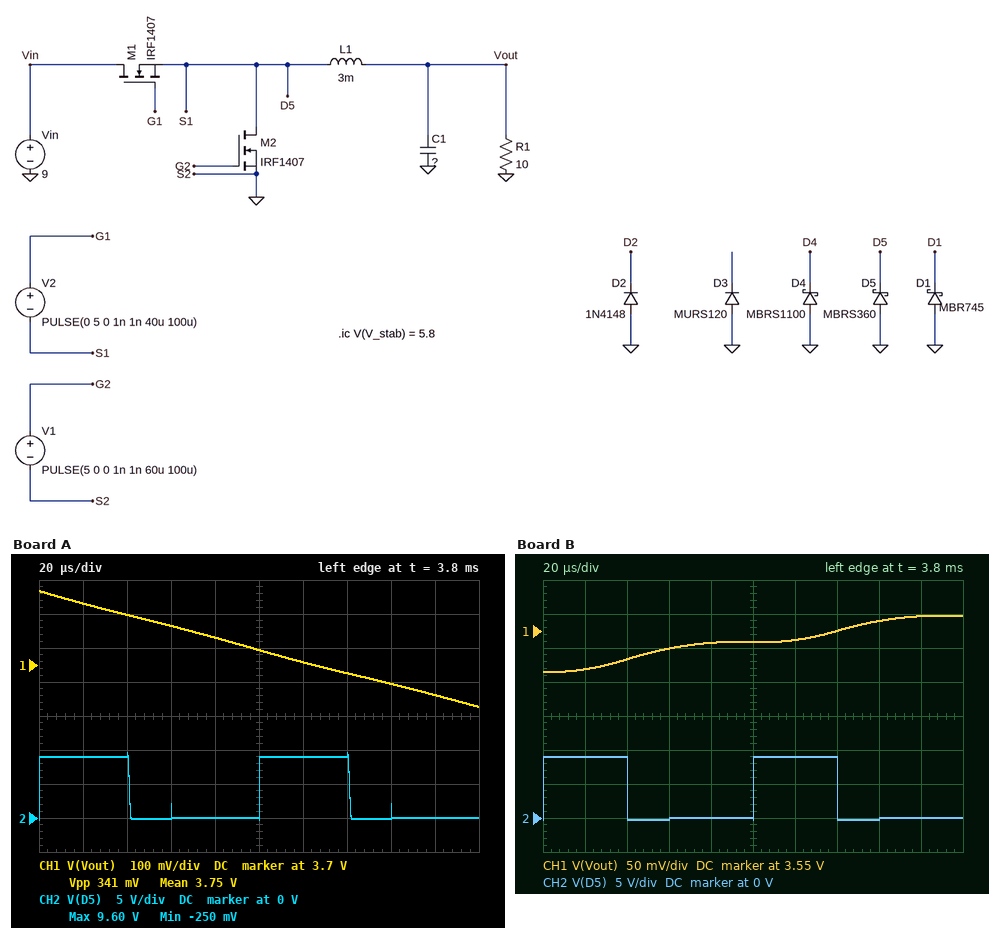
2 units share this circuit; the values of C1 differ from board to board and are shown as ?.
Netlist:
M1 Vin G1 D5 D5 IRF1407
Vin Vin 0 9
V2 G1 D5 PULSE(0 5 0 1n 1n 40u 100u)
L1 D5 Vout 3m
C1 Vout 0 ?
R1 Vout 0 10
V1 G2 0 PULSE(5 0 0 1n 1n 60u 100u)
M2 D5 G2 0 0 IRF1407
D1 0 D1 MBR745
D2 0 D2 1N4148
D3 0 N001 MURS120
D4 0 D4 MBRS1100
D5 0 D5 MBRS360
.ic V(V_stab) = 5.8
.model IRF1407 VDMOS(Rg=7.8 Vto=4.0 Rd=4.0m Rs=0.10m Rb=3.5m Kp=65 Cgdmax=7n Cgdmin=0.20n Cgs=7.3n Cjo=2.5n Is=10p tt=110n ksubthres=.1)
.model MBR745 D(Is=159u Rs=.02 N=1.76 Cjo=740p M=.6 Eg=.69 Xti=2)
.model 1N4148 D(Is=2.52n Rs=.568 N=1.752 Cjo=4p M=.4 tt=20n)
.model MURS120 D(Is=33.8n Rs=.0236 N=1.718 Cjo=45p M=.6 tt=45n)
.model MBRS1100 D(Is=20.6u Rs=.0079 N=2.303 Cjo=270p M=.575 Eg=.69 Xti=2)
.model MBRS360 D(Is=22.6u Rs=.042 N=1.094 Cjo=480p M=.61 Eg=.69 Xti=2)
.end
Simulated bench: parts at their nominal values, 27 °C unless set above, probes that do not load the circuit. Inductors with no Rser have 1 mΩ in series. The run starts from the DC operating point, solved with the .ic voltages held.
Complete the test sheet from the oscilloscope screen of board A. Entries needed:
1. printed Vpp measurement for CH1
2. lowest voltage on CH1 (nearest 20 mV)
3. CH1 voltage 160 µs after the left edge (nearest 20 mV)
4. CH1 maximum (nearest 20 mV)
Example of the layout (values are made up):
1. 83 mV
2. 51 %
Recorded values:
1. 341 mV
2. 3.58 V
3. 3.64 V
4. 3.92 V
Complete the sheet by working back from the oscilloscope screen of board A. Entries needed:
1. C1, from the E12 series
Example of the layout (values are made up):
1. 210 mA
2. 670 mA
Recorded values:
1. 220 µF
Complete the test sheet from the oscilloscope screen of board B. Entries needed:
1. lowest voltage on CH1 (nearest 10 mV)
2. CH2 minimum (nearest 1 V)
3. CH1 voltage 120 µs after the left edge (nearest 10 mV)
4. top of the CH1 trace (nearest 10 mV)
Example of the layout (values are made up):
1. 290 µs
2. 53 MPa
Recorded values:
1. 3.49 V
2. 0 V
3. 3.54 V
4. 3.57 V
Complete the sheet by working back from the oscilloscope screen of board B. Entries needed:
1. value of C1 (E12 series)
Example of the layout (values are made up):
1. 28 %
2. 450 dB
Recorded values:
1. 68 µF
